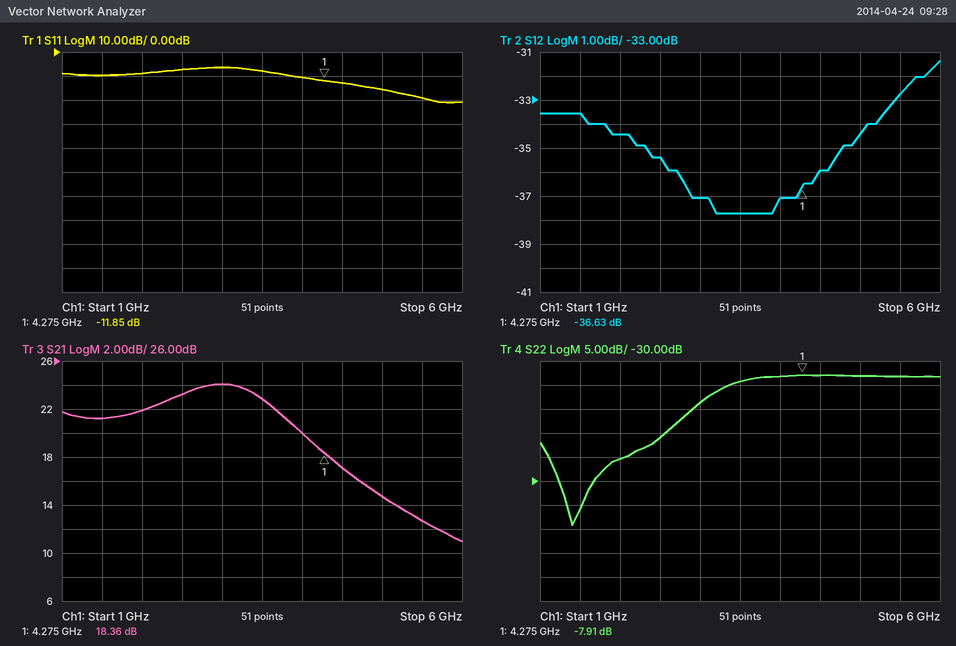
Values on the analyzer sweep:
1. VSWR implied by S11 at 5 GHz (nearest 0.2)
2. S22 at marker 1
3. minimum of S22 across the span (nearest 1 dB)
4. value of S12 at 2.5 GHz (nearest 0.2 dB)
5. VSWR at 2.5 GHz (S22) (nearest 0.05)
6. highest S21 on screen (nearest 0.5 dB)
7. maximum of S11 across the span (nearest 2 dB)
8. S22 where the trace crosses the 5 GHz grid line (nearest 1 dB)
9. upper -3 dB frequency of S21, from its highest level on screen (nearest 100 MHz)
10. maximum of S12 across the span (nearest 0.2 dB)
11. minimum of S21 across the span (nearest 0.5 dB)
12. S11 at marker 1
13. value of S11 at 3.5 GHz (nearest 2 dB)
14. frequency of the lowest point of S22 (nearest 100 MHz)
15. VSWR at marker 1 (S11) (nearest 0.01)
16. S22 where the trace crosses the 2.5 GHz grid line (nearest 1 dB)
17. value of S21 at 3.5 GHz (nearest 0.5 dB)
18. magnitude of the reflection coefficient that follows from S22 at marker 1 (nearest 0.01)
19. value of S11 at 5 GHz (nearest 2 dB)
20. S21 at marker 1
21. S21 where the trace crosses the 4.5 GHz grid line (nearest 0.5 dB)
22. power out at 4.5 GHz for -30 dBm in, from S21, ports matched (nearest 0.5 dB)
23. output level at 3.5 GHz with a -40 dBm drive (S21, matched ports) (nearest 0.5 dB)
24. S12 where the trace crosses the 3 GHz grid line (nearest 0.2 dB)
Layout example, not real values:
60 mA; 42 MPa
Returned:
1.4; -7.91 dB; -39 dB; -35.4 dB; 1.20; 24.0 dB; -6 dB; -8 dB; 3.8 GHz; -31.4 dB; 11.0 dB; -11.85 dB; -8 dB; 1.4 GHz; 1.69; -21 dB; 23.0 dB; 0.40; -16 dB; 18.36 dB; 17.0 dB; -13.0 dBm; -17.0 dBm; -37.0 dB
